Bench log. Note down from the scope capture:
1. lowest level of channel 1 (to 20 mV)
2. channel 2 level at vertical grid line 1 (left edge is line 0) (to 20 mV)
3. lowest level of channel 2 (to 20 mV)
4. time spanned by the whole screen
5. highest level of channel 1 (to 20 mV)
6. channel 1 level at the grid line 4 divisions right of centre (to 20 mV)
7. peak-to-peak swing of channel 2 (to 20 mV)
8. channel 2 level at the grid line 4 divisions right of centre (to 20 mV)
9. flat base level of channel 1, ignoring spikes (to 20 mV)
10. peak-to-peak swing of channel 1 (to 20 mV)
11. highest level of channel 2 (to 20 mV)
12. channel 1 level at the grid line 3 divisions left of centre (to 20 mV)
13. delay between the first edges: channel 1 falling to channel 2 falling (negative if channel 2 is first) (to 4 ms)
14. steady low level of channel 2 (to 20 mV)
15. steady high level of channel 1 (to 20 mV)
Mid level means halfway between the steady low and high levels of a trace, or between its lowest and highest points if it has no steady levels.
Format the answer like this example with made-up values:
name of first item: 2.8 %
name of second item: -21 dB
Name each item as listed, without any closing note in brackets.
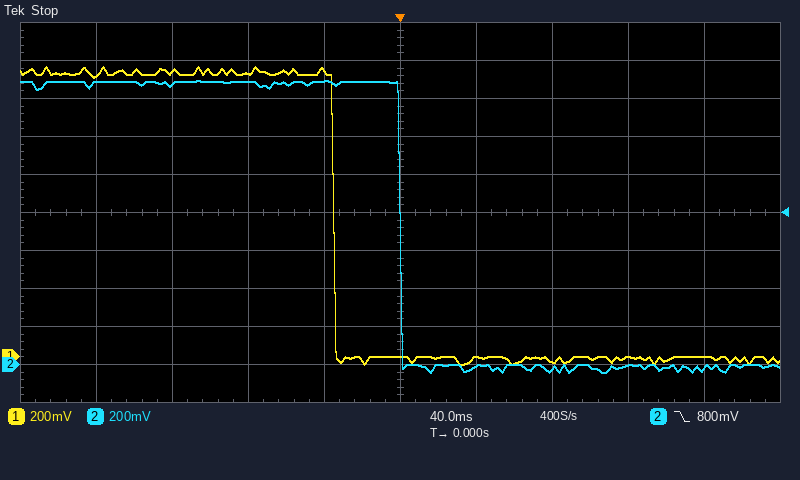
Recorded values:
lowest level of channel 1: -40 mV
channel 2 level at vertical grid line 1 (left edge is line 0): 1.48 V
lowest level of channel 2: -40 mV
time spanned by the whole screen: 400 ms
highest level of channel 1: 1.52 V
channel 1 level at the grid line 4 divisions right of centre: 0 mV
peak-to-peak swing of channel 2: 1.54 V
channel 2 level at the grid line 4 divisions right of centre: -20 mV
flat base level of channel 1, ignoring spikes: 0 mV
peak-to-peak swing of channel 1: 1.56 V
highest level of channel 2: 1.50 V
channel 1 level at the grid line 3 divisions left of centre: 1.50 V
delay between the first edges: channel 1 falling to channel 2 falling (negative if channel 2 is first): +36 ms
steady low level of channel 2: 0 mV
steady high level of channel 1: 1.48 V
